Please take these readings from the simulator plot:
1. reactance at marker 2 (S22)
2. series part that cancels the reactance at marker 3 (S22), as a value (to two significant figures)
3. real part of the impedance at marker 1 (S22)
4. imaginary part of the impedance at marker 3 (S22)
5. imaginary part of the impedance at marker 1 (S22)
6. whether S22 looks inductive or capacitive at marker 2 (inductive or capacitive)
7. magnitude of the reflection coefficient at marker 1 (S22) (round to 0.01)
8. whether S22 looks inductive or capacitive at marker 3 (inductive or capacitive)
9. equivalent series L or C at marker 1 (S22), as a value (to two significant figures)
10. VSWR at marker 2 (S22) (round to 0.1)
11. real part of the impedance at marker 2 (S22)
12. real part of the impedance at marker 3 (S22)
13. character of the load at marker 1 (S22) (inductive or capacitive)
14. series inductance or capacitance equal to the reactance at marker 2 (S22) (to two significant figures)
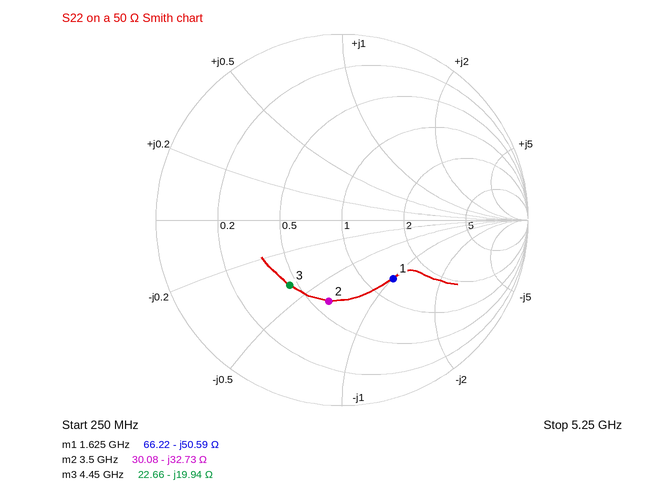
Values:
-32.73 Ω
710 pH
66.22 Ω
-19.94 Ω
-50.59 Ω
capacitive
0.42
capacitive
1.9 pF
2.6
30.08 Ω
22.66 Ω
capacitive
1.4 pF
